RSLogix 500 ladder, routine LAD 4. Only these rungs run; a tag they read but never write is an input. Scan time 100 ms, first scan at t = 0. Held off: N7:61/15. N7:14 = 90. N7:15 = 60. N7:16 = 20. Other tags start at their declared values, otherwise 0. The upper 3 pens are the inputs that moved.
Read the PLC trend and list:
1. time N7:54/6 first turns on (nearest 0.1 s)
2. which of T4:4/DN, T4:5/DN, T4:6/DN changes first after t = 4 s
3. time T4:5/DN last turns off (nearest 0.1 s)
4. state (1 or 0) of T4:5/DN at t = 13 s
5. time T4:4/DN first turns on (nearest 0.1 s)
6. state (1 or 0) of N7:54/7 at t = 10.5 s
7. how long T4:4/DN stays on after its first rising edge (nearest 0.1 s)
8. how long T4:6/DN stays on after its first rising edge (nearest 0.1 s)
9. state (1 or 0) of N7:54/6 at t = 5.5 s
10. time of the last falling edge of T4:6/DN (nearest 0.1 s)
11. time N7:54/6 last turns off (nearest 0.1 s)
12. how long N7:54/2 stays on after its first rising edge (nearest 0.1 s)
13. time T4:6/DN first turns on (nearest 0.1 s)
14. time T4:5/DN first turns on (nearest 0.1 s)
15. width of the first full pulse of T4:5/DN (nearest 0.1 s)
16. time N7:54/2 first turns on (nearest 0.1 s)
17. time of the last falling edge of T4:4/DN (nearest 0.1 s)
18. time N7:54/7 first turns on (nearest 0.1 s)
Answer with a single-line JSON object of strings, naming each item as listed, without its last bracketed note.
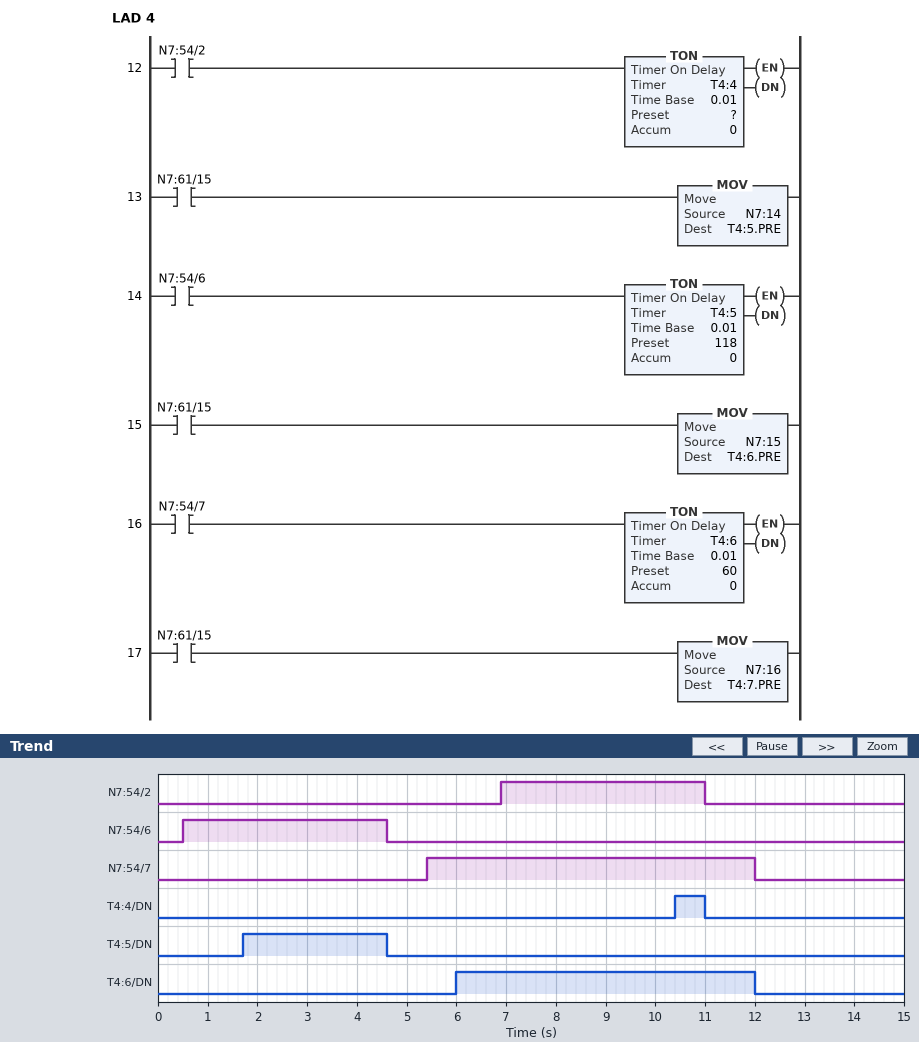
{"time N7:54/6 first turns on": "0.5 s", "which of T4:4/DN, T4:5/DN, T4:6/DN changes first after t = 4 s": "T4:5/DN", "time T4:5/DN last turns off": "4.6 s", "state (1 or 0) of T4:5/DN at t = 13 s": "0", "time T4:4/DN first turns on": "10.4 s", "state (1 or 0) of N7:54/7 at t = 10.5 s": "1", "how long T4:4/DN stays on after its first rising edge": "0.6 s", "how long T4:6/DN stays on after its first rising edge": "6.0 s", "state (1 or 0) of N7:54/6 at t = 5.5 s": "0", "time of the last falling edge of T4:6/DN": "12.0 s", "time N7:54/6 last turns off": "4.6 s", "how long N7:54/2 stays on after its first rising edge": "4.1 s", "time T4:6/DN first turns on": "6.0 s", "time T4:5/DN first turns on": "1.7 s", "width of the first full pulse of T4:5/DN": "2.9 s", "time N7:54/2 first turns on": "6.9 s", "time of the last falling edge of T4:4/DN": "11.0 s", "time N7:54/7 first turns on": "5.4 s"}
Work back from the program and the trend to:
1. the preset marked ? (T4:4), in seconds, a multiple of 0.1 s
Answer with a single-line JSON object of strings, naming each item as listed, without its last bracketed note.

{"the preset marked ? (T4:4), in seconds, a multiple of 0.1 s": "3.5 s"}
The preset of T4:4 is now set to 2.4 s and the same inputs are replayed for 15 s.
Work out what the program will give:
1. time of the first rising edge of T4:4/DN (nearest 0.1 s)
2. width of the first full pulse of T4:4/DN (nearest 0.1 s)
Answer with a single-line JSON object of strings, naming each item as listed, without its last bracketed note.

{"time of the first rising edge of T4:4/DN": "9.3 s", "width of the first full pulse of T4:4/DN": "1.7 s"}
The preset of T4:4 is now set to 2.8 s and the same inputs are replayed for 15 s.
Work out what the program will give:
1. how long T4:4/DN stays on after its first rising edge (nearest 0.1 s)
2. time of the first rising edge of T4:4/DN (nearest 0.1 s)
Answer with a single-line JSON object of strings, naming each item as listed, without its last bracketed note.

{"how long T4:4/DN stays on after its first rising edge": "1.3 s", "time of the first rising edge of T4:4/DN": "9.7 s"}
